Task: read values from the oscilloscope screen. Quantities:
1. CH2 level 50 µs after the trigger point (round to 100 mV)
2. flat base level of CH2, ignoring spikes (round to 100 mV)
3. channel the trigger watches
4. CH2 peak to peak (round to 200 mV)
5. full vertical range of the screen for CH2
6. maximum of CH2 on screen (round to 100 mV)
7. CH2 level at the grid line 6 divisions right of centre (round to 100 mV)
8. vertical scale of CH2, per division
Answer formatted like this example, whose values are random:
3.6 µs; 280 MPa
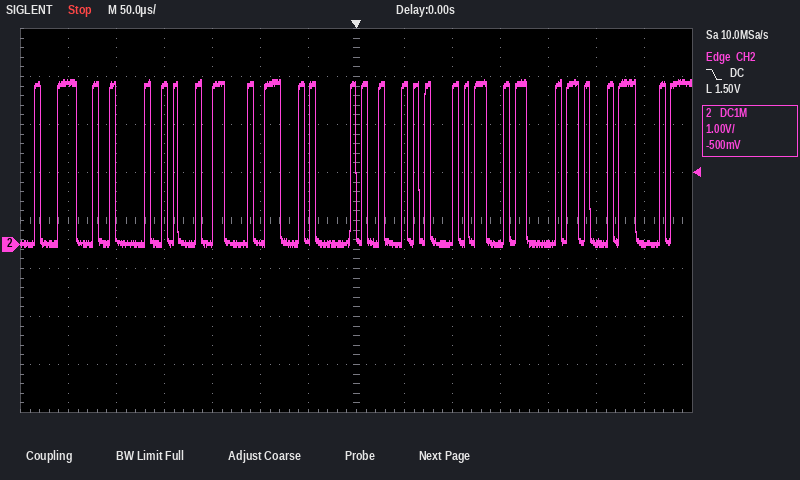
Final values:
3.3 V; 0.0 V; CH2; 3.4 V; 8 V; 3.4 V; 0.0 V; 1 V
